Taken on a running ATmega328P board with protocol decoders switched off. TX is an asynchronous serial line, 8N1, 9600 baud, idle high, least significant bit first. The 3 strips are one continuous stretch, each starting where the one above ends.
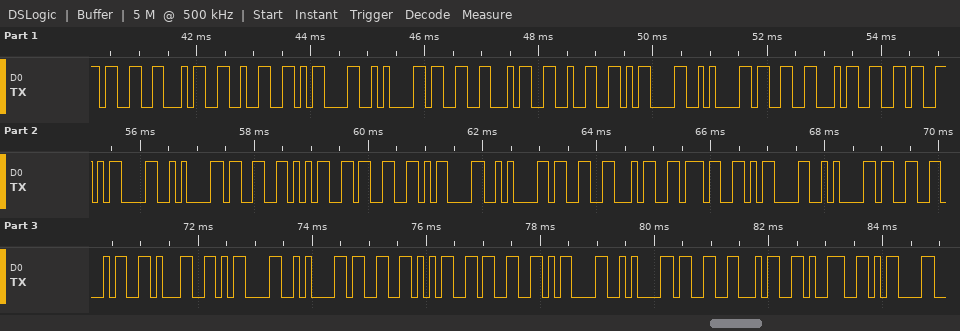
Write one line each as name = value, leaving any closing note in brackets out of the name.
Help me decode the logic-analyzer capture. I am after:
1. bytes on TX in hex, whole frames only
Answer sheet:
bytes on TX in hex, whole frames only = 33 34 32 0D 0A 33 34 32 0D 0A 33 34 36 0D 0A 33 35 33 0D 0A 33 34 37 0D 0A 33 34 31 0D 0A 33 35 33 0D 0A 33 34 39 0D
